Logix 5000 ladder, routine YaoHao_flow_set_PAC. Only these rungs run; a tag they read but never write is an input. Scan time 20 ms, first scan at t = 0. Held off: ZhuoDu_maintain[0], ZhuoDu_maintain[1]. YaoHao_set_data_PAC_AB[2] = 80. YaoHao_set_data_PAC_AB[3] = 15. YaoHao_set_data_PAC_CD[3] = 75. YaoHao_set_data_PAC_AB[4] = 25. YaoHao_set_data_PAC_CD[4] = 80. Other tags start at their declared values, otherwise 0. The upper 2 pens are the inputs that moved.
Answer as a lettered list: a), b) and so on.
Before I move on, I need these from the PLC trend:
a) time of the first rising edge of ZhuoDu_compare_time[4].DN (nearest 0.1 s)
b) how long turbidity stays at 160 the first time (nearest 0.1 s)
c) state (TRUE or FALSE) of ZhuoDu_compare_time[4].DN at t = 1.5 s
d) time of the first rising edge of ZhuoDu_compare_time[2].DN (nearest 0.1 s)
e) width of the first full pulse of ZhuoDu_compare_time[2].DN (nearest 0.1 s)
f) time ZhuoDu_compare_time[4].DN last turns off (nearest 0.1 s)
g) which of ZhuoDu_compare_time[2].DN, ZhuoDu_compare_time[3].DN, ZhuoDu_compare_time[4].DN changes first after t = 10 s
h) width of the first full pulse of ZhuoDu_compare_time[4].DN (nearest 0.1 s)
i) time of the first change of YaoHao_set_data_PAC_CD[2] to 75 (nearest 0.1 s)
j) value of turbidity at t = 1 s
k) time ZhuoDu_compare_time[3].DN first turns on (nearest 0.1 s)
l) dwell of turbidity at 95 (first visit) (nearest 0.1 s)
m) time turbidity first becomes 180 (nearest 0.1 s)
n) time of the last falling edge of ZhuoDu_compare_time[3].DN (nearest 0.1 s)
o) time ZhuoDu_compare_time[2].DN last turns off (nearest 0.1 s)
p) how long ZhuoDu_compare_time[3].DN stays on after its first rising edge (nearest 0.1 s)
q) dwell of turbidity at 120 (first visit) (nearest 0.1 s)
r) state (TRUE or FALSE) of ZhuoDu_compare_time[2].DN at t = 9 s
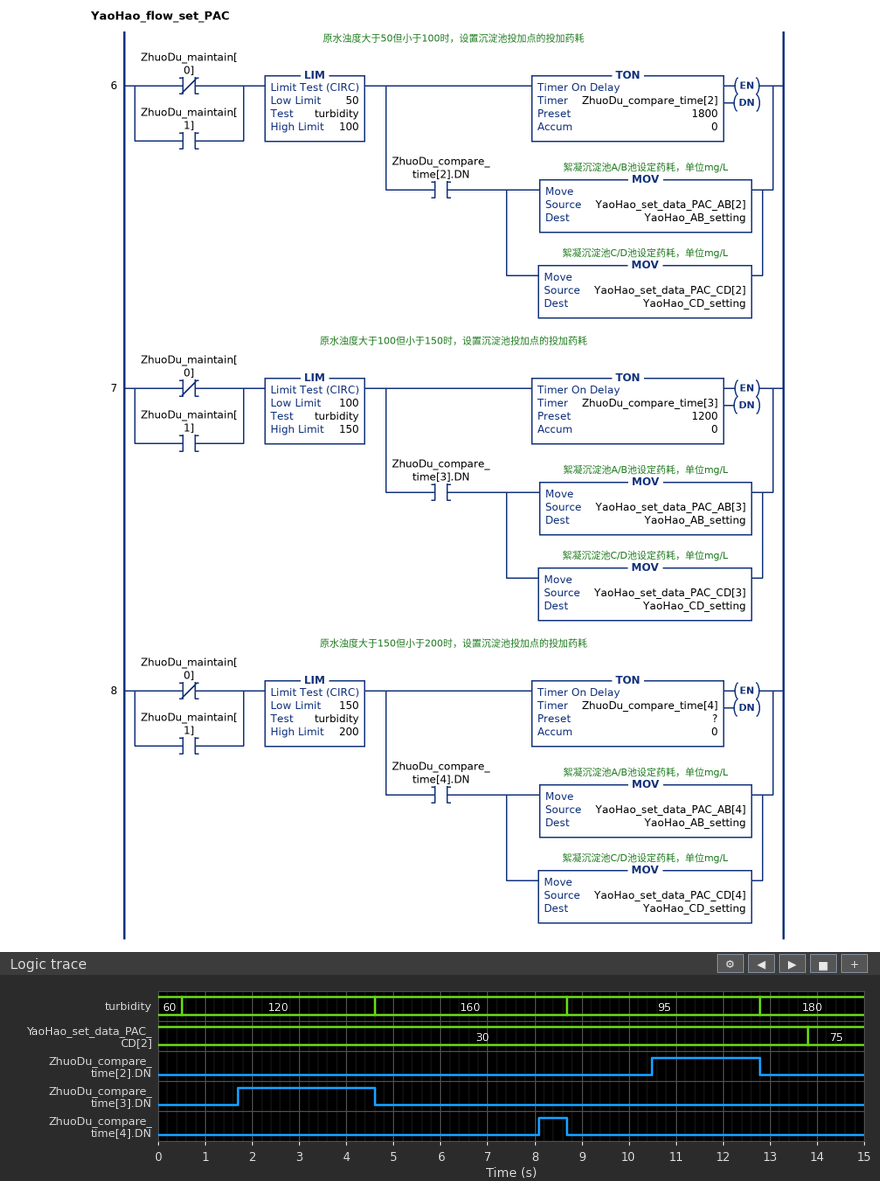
a) 8.1 s
b) 4.1 s
c) FALSE
d) 10.5 s
e) 2.3 s
f) 8.7 s
g) ZhuoDu_compare_time[2].DN
h) 0.6 s
i) 13.8 s
j) 120
k) 1.7 s
l) 4.1 s
m) 12.8 s
n) 4.6 s
o) 12.8 s
p) 2.9 s
q) 4.1 s
r) FALSE
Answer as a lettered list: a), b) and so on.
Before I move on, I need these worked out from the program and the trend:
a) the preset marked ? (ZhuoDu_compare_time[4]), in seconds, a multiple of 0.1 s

a) 3.5 s
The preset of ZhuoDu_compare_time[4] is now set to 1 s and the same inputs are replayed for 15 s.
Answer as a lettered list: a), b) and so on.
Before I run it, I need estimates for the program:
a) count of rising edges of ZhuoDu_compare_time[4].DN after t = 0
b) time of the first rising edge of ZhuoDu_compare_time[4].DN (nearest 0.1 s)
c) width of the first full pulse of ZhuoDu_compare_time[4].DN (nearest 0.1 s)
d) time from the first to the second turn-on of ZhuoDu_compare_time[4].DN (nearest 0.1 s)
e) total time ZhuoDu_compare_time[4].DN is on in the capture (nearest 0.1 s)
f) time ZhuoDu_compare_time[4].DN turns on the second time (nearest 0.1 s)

a) 2
b) 5.6 s
c) 3.1 s
d) 8.2 s
e) 4.3 s
f) 13.8 s
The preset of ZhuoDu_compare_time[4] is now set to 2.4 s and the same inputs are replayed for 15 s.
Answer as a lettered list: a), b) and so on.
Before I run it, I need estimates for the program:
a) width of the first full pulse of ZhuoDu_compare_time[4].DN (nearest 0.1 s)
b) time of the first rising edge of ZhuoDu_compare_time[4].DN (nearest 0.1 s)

a) 1.7 s
b) 7.0 s
